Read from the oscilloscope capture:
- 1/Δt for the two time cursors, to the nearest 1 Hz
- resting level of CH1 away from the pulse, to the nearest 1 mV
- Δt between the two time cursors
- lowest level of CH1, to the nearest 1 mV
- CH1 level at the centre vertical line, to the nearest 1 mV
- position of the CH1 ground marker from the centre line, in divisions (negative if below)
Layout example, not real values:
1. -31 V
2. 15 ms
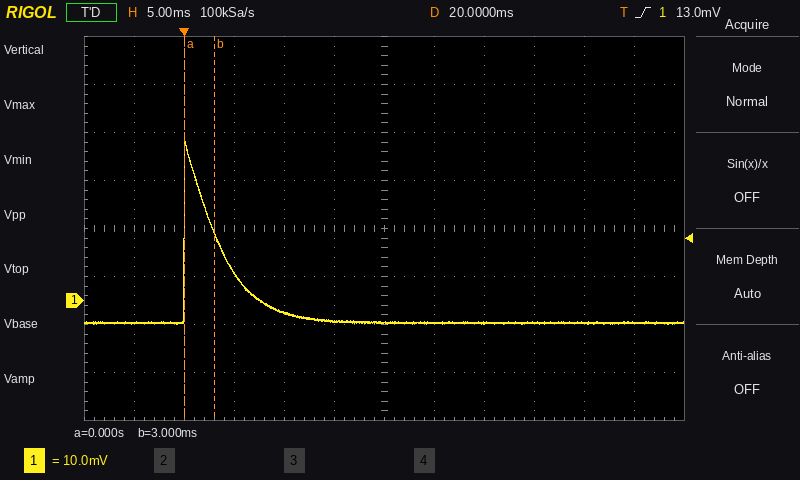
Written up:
1. 333 Hz
2. -5 mV
3. 3.0 ms
4. -5 mV
5. -5 mV
6. -1.5 div
